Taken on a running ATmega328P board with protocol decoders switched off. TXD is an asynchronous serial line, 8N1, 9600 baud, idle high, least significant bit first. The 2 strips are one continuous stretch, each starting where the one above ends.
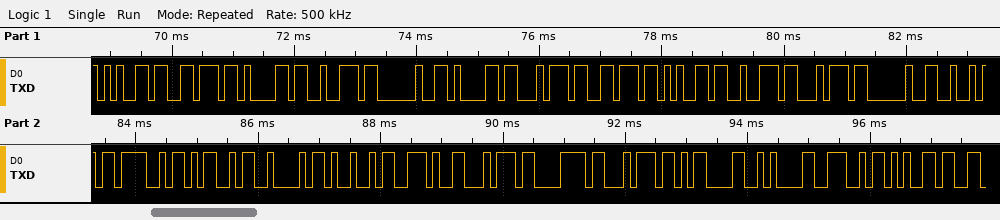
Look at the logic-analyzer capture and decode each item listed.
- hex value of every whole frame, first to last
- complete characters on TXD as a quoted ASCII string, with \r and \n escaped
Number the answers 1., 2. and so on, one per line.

1. 65 76 61 72 20 61 74 76 65 72 74 20 52 4F 4D 42 49 2E 74 78 74 0D 0A 4E 65
2. "evar atvert ROMBI.txt\r\nNe"
